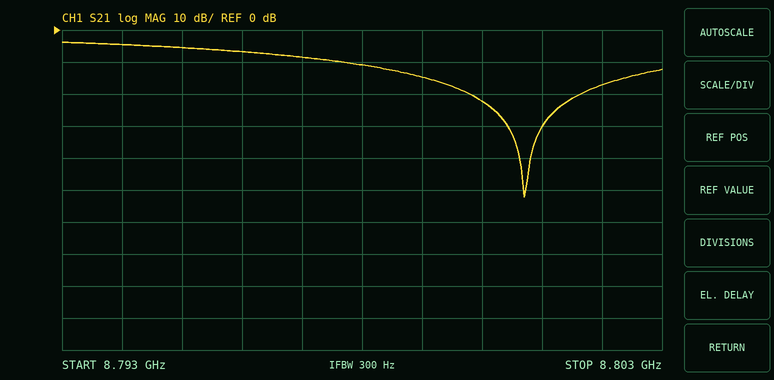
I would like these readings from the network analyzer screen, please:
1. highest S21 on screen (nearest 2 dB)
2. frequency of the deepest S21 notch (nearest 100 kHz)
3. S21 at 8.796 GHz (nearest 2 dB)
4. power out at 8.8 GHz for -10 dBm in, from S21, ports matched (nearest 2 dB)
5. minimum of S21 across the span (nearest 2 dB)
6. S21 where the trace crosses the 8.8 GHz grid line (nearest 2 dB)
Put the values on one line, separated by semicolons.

-4 dB; 8.8007 GHz; -6 dB; -32 dBm; -52 dB; -22 dB
